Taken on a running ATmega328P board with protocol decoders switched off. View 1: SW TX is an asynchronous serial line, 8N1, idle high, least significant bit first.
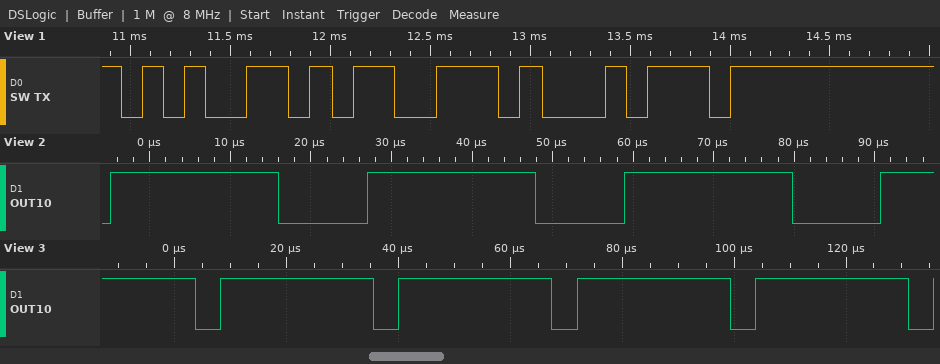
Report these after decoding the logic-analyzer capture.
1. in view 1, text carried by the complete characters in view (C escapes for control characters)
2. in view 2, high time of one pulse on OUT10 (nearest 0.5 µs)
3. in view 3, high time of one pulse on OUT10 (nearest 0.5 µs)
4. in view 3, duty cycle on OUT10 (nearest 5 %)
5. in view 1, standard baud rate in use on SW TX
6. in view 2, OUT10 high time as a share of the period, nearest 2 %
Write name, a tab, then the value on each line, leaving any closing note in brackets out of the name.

in view 1, text carried by the complete characters in view	"est"
in view 2, high time of one pulse on OUT10	21.0 µs
in view 3, high time of one pulse on OUT10	27.5 µs
in view 3, duty cycle on OUT10	85 %
in view 1, standard baud rate in use on SW TX	9600 baud
in view 2, OUT10 high time as a share of the period, nearest 2 %	66 %
